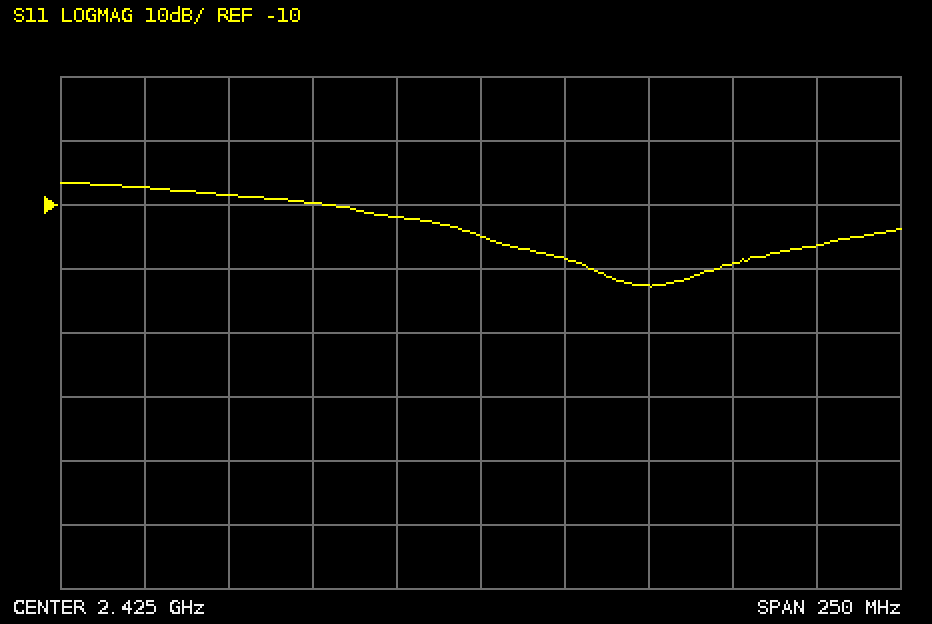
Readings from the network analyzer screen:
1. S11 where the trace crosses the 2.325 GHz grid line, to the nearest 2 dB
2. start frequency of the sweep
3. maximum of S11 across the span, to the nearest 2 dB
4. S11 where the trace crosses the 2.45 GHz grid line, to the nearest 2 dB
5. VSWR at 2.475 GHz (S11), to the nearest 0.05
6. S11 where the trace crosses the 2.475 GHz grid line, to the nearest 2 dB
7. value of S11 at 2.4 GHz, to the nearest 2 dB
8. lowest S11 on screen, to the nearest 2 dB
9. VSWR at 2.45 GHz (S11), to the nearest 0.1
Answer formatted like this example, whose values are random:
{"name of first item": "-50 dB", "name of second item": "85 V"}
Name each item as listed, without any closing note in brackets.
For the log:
{"S11 where the trace crosses the 2.325 GHz grid line, to the nearest 2 dB": "-8 dB", "start frequency of the sweep": "2.3 GHz", "maximum of S11 across the span, to the nearest 2 dB": "-6 dB", "S11 where the trace crosses the 2.45 GHz grid line, to the nearest 2 dB": "-18 dB", "VSWR at 2.475 GHz (S11), to the nearest 0.05": "1.15", "S11 where the trace crosses the 2.475 GHz grid line, to the nearest 2 dB": "-22 dB", "value of S11 at 2.4 GHz, to the nearest 2 dB": "-12 dB", "lowest S11 on screen, to the nearest 2 dB": "-22 dB", "VSWR at 2.45 GHz (S11), to the nearest 0.1": "1.3"}
